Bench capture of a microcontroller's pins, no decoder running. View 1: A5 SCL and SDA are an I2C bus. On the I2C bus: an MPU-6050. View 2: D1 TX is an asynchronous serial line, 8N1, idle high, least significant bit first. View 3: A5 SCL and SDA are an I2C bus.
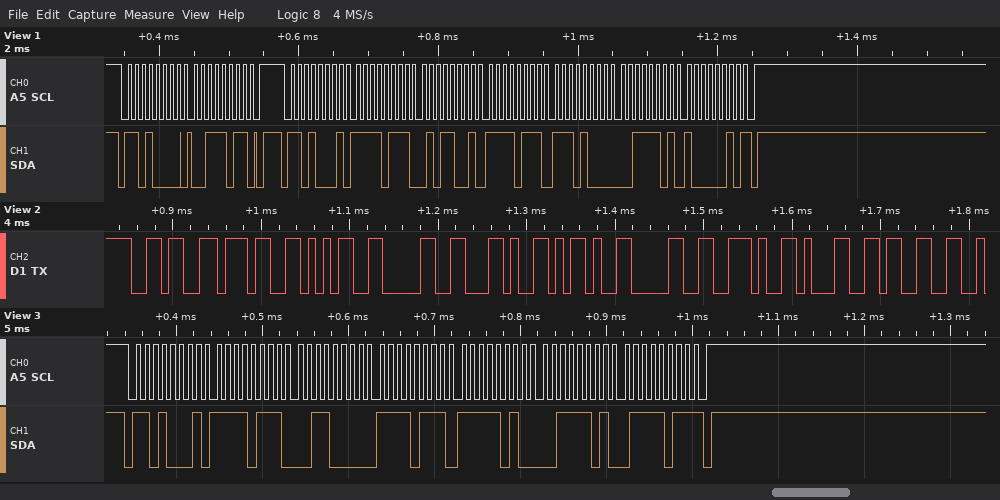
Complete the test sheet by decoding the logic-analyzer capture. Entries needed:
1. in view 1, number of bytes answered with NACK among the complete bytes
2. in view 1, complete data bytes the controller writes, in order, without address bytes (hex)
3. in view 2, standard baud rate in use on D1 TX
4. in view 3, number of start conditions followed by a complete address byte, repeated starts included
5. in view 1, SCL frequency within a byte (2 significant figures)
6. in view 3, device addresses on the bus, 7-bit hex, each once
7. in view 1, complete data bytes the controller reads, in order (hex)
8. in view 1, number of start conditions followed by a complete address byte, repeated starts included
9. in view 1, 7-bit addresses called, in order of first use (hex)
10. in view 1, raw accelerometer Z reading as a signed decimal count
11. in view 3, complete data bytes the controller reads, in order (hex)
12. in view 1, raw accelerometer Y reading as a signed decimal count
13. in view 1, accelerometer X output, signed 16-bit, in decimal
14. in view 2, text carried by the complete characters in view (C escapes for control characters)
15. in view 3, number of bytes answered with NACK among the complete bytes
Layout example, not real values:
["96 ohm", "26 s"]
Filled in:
["1", "3B", "115200 baud", "1", "100 kHz", "0x68", "F7 59 F7 E8 3D 82", "2", "0x68", "15746", "F7 30 F7 FA 3D 7B", "-2072", "-2215", "\"6750,-0.13\"", "1"]
